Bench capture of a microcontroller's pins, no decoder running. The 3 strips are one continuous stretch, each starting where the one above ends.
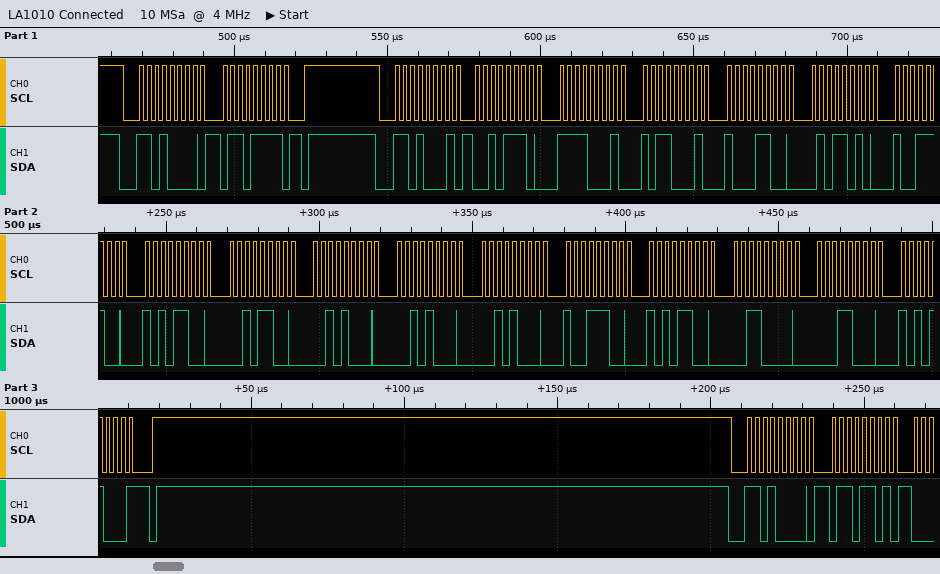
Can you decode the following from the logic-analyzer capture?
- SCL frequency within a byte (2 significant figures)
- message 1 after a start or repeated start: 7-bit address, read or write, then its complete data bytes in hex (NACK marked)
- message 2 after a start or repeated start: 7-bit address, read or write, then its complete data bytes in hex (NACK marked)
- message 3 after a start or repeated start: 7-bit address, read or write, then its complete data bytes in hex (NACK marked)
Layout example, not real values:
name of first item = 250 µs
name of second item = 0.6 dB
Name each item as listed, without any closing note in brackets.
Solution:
SCL frequency within a byte = 400 kHz
message 1 after a start or repeated start: 7-bit address, read or write, then its complete data bytes in hex = 0x68 write: 6F
message 2 after a start or repeated start: 7-bit address, read or write, then its complete data bytes in hex = 0x68 read: 2E F1 B1 8C 5A 9C AC 2C 28 28 28 9C AC 30 18 A8 NACK
message 3 after a start or repeated start: 7-bit address, read or write, then its complete data bytes in hex = 0x68 write: 6D
